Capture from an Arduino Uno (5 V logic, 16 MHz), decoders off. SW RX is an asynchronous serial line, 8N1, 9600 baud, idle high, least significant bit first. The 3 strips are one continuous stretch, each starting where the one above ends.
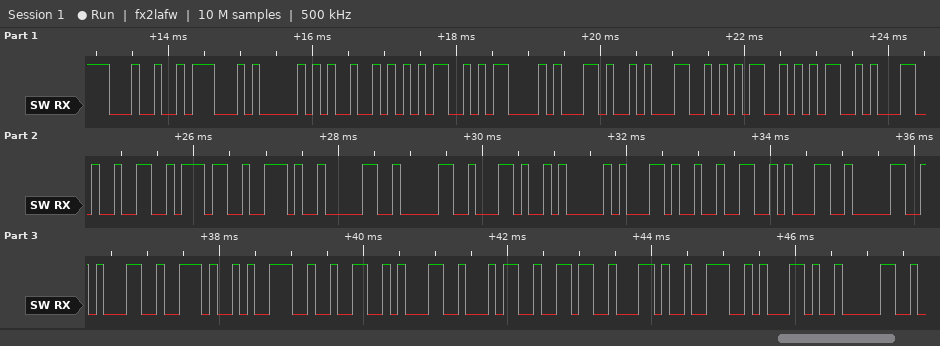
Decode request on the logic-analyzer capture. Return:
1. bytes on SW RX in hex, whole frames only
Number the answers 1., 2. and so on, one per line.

1. 0x24 0x47 0x50 0x52 0x4D 0x43 0x2C 0x31 0x35 0x35 0x31 0x32 0x37 0x2E 0x30 0x30 0x2C 0x41 0x2C 0x32 0x31 0x30 0x31 0x2E 0x39 0x32 0x31 0x34 0x36 0x2C 0x4E 0x2C 0x30
